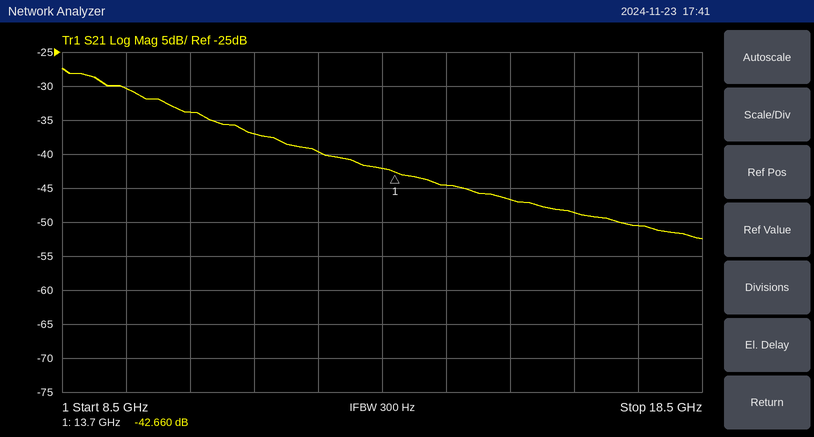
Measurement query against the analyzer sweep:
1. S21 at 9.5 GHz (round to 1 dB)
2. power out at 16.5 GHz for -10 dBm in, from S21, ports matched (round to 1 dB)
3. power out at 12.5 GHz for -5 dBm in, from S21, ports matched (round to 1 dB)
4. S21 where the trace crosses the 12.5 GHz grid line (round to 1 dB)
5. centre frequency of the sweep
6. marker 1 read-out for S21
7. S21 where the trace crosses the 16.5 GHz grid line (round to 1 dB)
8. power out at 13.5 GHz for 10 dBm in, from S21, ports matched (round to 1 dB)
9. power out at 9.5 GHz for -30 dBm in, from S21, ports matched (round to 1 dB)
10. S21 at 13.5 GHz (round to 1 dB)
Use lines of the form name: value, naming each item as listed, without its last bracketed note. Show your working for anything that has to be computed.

S21 at 9.5 GHz: -30 dB
power out at 16.5 GHz for -10 dBm in, from S21, ports matched: -10 dBm + (-49 dB) = -59 dBm
power out at 12.5 GHz for -5 dBm in, from S21, ports matched: -5 dBm + (-40 dB) = -45 dBm
S21 where the trace crosses the 12.5 GHz grid line: -40 dB
centre frequency of the sweep: 13.5 GHz
marker 1 read-out for S21: -42.660 dB
S21 where the trace crosses the 16.5 GHz grid line: -49 dB
power out at 13.5 GHz for 10 dBm in, from S21, ports matched: 10 dBm + (-42 dB) = -32 dBm
power out at 9.5 GHz for -30 dBm in, from S21, ports matched: -30 dBm + (-30 dB) = -60 dBm
S21 at 13.5 GHz: -42 dB
